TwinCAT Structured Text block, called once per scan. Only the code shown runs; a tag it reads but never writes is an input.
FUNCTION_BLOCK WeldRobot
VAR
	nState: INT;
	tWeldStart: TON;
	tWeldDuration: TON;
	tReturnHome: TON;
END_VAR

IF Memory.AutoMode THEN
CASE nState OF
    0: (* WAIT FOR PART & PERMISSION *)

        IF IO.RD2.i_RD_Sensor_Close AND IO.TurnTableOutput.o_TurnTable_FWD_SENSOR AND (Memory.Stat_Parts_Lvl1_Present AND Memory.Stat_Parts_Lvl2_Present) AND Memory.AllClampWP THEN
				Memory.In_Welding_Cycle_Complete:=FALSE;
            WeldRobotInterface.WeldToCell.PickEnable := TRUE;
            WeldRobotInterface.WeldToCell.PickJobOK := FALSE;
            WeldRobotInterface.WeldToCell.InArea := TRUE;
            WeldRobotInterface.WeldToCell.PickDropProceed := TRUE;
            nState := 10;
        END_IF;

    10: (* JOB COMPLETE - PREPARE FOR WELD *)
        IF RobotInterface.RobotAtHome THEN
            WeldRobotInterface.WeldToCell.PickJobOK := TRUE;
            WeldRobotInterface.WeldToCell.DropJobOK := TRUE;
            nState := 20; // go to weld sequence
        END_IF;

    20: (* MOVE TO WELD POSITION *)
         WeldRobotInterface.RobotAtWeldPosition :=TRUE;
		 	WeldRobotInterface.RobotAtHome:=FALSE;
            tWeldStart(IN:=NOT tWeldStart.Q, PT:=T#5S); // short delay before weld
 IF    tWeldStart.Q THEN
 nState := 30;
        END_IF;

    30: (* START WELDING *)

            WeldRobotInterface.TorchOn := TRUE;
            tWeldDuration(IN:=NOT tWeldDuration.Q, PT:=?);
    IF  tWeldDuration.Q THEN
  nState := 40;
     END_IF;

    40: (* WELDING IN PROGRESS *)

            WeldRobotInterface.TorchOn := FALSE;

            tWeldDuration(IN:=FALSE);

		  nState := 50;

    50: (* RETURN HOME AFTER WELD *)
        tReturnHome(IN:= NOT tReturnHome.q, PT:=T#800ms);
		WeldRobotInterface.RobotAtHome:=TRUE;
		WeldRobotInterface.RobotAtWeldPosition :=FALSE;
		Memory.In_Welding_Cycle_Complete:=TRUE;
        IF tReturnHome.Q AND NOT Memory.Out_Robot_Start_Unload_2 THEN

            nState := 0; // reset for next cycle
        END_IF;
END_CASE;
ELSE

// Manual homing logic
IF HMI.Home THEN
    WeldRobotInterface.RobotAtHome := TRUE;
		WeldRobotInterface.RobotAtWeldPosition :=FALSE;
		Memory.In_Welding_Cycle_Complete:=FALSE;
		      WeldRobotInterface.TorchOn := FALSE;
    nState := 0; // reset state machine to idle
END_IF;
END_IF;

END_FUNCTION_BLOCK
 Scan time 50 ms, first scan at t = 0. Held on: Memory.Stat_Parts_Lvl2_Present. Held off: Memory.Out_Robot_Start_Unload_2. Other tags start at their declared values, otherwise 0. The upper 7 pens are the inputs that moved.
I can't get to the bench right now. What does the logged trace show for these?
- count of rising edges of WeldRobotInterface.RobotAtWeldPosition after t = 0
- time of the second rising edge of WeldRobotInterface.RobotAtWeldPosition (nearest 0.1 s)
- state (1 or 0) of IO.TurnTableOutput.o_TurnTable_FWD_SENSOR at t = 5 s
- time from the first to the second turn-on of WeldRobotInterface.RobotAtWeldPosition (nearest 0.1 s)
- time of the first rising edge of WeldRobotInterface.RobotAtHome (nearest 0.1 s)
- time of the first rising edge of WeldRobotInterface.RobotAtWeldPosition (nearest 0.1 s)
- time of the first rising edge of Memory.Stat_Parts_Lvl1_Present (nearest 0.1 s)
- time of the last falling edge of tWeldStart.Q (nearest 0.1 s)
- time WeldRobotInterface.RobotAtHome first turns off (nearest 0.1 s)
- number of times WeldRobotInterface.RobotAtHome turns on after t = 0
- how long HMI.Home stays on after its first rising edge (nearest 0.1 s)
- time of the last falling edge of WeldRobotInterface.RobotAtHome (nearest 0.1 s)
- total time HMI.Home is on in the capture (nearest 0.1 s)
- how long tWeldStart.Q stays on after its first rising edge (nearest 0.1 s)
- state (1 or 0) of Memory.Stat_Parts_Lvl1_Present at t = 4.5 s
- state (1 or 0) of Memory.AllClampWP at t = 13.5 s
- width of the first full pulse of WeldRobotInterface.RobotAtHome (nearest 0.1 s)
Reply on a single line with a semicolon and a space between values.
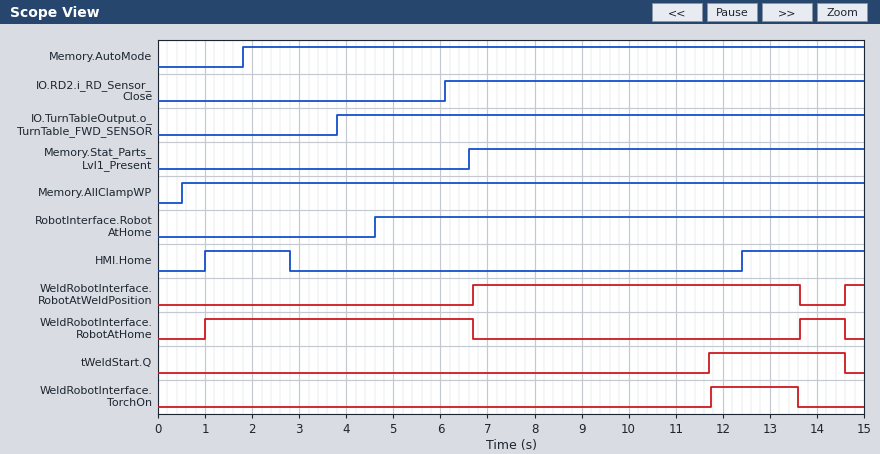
2; 14.6 s; 1; 7.9 s; 1.0 s; 6.7 s; 6.6 s; 14.6 s; 6.7 s; 2; 1.8 s; 14.6 s; 4.4 s; 2.9 s; 0; 1; 5.7 s
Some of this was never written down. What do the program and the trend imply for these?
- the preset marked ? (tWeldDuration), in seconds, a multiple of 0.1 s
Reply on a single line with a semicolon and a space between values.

1.8 s
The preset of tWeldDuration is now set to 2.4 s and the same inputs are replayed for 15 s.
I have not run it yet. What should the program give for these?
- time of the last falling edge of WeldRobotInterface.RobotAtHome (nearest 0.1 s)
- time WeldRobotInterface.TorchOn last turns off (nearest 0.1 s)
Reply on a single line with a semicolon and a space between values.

6.7 s; 14.2 s
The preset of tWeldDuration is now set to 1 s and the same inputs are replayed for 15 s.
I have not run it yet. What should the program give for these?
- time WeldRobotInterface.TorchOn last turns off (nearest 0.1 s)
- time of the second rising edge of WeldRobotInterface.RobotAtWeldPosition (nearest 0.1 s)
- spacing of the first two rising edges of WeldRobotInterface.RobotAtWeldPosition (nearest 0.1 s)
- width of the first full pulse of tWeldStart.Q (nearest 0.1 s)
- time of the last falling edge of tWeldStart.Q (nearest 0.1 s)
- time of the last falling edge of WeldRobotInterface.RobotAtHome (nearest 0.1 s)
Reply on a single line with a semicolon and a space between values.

12.8 s; 13.8 s; 7.1 s; 2.1 s; 13.8 s; 13.8 s
